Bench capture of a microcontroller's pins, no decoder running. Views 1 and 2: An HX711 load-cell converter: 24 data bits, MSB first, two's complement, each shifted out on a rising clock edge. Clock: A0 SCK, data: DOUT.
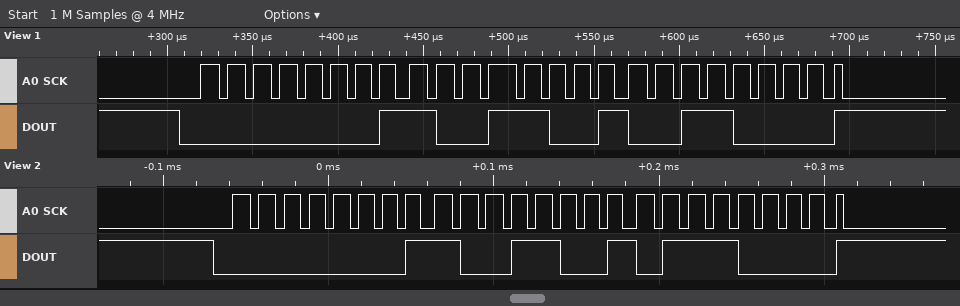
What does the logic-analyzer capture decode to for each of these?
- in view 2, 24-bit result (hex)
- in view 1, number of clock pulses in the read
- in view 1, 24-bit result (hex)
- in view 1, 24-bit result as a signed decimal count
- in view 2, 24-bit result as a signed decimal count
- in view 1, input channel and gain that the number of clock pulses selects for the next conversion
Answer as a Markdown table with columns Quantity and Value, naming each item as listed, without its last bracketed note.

| Quantity | Value |
|---|---|
| in view 2, 24-bit result | 0x019970 |
| in view 1, number of clock pulses in the read | 25 |
| in view 1, 24-bit result | 0x019930 |
| in view 1, 24-bit result as a signed decimal count | 104752 |
| in view 2, 24-bit result as a signed decimal count | 104816 |
| in view 1, input channel and gain that the number of clock pulses selects for the next conversion | channel A, gain 128 |
